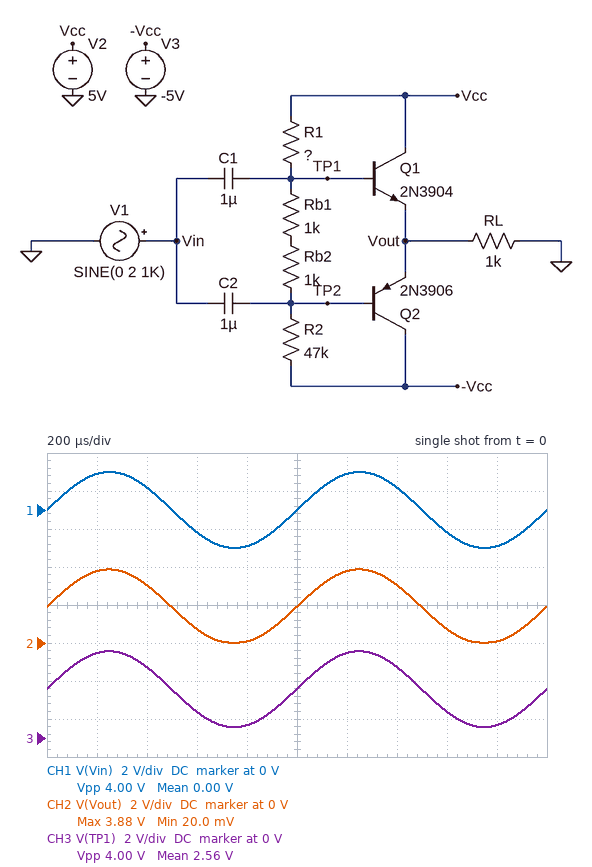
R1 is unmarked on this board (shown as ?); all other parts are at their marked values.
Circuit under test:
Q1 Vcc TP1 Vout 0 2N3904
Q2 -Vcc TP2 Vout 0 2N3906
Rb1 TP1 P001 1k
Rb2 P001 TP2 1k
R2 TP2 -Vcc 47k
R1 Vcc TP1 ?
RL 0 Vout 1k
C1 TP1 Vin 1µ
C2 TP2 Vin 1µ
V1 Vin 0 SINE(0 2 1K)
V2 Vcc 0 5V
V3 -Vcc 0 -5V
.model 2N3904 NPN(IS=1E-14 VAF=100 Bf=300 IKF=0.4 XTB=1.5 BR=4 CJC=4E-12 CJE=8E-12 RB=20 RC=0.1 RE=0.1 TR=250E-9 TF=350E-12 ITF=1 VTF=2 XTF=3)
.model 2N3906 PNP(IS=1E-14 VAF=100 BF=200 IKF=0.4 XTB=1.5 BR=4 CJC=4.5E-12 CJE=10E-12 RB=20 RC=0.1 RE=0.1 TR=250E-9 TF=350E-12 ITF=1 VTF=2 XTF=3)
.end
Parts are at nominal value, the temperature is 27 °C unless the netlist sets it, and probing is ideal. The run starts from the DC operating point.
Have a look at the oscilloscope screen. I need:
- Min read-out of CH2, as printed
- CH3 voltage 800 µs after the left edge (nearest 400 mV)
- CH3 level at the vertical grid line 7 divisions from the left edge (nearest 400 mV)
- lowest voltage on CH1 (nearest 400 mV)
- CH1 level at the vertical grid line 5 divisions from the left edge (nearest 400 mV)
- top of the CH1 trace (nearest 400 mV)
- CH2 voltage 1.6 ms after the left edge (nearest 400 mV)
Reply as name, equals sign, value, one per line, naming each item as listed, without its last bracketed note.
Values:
Min read-out of CH2, as printed = 20.0 mV
CH3 voltage 800 µs after the left edge = 800 mV
CH3 level at the vertical grid line 7 divisions from the left edge = 3.6 V
lowest voltage on CH1 = -2.0 V
CH1 level at the vertical grid line 5 divisions from the left edge = 0 V
top of the CH1 trace = 2.0 V
CH2 voltage 1.6 ms after the left edge = 800 mV
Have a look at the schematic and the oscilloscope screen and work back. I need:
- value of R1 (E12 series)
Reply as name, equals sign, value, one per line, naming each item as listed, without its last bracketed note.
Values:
value of R1 = 15 kΩ
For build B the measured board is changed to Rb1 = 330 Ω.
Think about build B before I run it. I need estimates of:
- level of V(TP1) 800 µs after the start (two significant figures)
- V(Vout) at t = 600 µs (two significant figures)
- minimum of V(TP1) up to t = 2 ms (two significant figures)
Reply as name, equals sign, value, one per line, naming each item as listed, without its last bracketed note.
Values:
level of V(TP1) 800 µs after the start = 650 mV
V(Vout) at t = 600 µs = 710 mV
minimum of V(TP1) up to t = 2 ms = 550 mV
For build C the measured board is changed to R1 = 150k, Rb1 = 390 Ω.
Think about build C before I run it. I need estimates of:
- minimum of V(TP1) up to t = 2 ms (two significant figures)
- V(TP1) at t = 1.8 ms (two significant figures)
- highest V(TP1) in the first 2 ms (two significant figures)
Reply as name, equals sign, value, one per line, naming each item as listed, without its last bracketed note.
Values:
minimum of V(TP1) up to t = 2 ms = -4.3 V
V(TP1) at t = 1.8 ms = -4.2 V
highest V(TP1) in the first 2 ms = -270 mV
